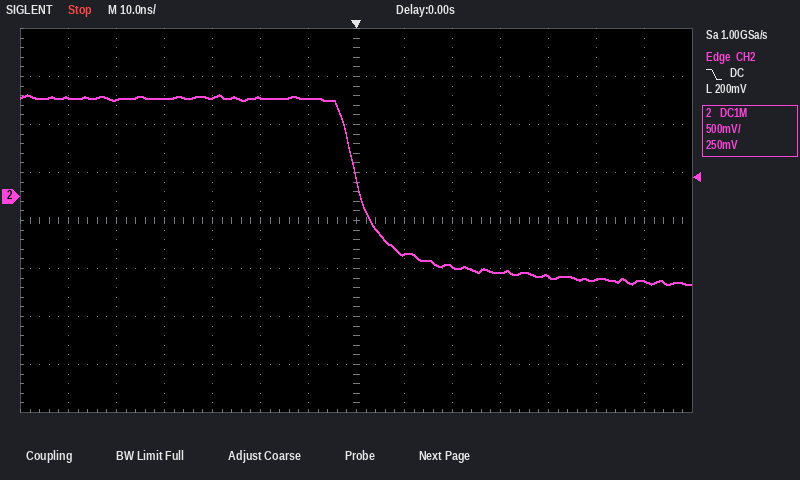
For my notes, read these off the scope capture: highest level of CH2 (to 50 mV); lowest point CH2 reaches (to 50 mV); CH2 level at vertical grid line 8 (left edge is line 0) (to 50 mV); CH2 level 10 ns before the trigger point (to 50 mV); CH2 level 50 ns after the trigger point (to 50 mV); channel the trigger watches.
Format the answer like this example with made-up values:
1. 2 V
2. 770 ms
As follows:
1. 1.05 V
2. -900 mV
3. -600 mV
4. 1.00 V
5. -850 mV
6. CH2
